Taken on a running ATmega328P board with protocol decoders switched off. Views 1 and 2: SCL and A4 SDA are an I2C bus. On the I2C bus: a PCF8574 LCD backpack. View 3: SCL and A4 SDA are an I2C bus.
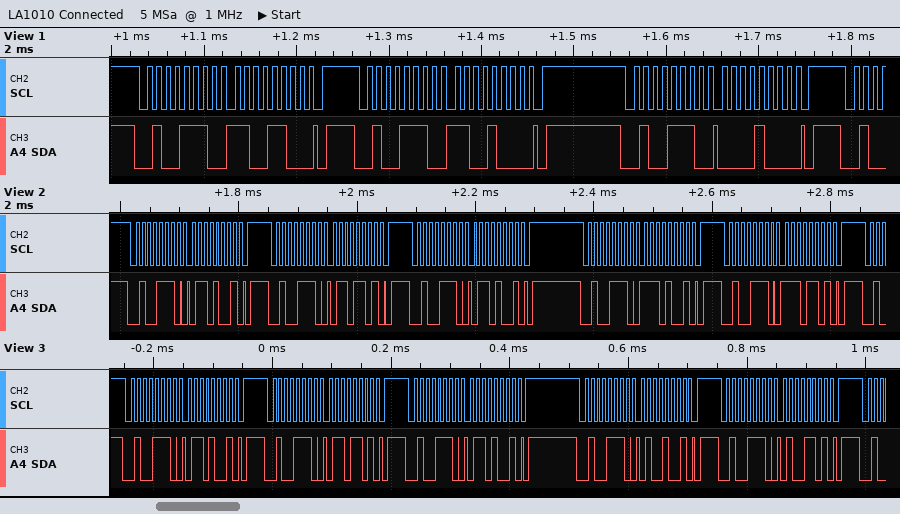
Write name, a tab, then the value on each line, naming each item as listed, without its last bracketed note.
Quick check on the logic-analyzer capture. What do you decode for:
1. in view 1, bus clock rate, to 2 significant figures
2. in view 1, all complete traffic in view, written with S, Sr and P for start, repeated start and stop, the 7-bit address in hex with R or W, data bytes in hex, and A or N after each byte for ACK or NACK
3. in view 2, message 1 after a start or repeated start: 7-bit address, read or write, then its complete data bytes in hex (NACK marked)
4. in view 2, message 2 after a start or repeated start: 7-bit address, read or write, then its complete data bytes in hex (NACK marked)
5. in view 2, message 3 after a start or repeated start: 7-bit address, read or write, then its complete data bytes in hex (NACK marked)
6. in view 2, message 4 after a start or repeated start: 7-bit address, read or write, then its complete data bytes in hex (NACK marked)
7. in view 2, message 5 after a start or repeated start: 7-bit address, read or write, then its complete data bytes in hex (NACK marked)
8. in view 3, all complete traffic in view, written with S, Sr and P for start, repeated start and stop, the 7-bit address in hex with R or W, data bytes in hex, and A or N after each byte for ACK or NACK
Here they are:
in view 1, bus clock rate, to 2 significant figures	100 kHz
in view 1, all complete traffic in view, written with S, Sr and P for start, repeated start and stop, the 7-bit address in hex with R or W, data bytes in hex, and A or N after each byte for ACK or NACK	S 27W A CC A P S 27W A C8 A P S 27W A 08 A P
in view 2, message 1 after a start or repeated start: 7-bit address, read or write, then its complete data bytes in hex	0x27 write: 69
in view 2, message 2 after a start or repeated start: 7-bit address, read or write, then its complete data bytes in hex	0x27 write: 6D
in view 2, message 3 after a start or repeated start: 7-bit address, read or write, then its complete data bytes in hex	0x27 write: 69
in view 2, message 4 after a start or repeated start: 7-bit address, read or write, then its complete data bytes in hex	0x27 write: E9
in view 2, message 5 after a start or repeated start: 7-bit address, read or write, then its complete data bytes in hex	0x27 write: ED
in view 3, all complete traffic in view, written with S, Sr and P for start, repeated start and stop, the 7-bit address in hex with R or W, data bytes in hex, and A or N after each byte for ACK or NACK	S 27W A 69 A P S 27W A 6D A P S 27W A 69 A P S 27W A 49 A P S 27W A 4D A P
